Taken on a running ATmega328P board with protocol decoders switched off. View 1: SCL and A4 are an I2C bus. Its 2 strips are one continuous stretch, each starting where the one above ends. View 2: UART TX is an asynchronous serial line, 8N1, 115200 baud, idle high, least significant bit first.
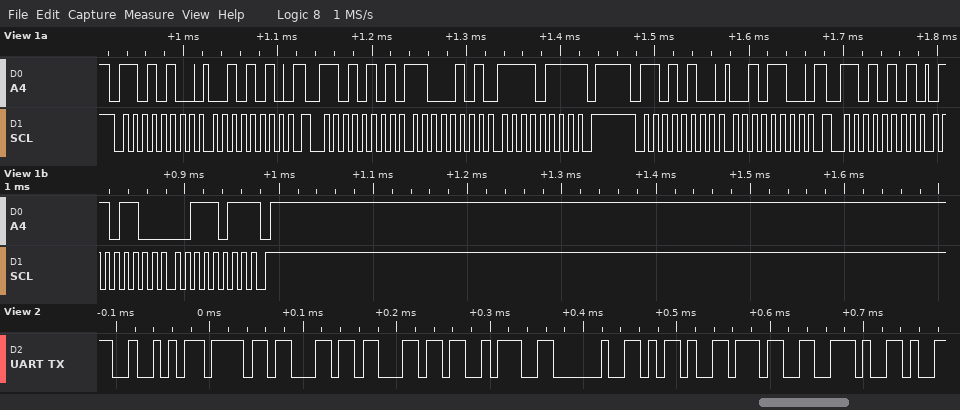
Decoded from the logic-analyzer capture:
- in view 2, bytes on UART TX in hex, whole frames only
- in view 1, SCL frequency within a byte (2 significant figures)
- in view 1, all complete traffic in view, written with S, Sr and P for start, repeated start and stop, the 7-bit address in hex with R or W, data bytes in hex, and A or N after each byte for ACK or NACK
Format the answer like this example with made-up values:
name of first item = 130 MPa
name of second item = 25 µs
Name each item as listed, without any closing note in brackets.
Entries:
in view 2, bytes on UART TX in hex, whole frames only = 0x52 0x6F 0x6C 0x6C 0x3A 0x20 0x2D 0x37 0x2E
in view 1, SCL frequency within a byte = 100 kHz
in view 1, all complete traffic in view, written with S, Sr and P for start, repeated start and stop, the 7-bit address in hex with R or W, data bytes in hex, and A or N after each byte for ACK or NACK = S 6AW A 2A A Sr 6AR A C5 A F7 N P S 6AW A 2C A Sr 6AR A 6C A 3B N P
